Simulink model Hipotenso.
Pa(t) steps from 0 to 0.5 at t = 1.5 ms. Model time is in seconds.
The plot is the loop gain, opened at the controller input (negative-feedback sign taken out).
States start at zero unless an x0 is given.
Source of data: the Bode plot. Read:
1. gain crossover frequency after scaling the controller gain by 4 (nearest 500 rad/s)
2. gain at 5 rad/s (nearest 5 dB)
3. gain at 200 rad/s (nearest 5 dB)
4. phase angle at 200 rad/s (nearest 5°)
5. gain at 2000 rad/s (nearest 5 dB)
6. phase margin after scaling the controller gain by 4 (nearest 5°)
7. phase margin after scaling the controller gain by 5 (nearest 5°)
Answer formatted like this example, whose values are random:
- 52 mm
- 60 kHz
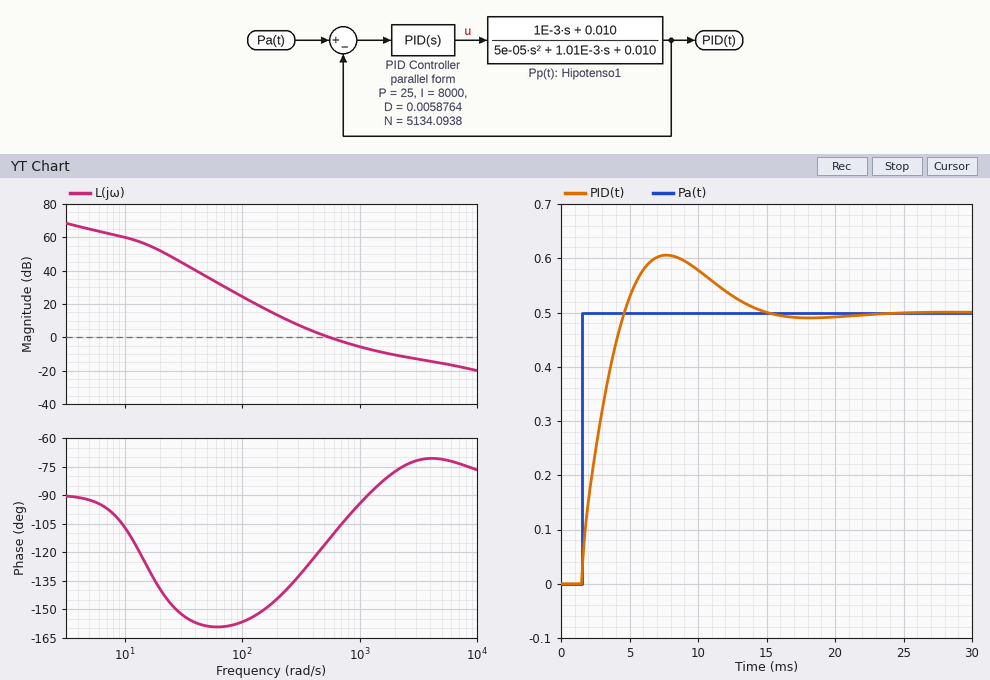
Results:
- 2500 rad/s
- 65 dB
- 15 dB
- -145°
- -10 dB
- 105°
- 110°
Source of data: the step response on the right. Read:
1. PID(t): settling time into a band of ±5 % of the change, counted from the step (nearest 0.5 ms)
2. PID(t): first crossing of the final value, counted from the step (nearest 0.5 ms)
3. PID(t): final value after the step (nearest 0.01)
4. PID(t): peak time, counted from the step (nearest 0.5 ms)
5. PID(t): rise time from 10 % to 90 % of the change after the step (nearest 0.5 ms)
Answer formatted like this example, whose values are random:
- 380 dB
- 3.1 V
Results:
- 11.5 ms
- 3.0 ms
- 0.50
- 6.0 ms
- 2.5 ms
